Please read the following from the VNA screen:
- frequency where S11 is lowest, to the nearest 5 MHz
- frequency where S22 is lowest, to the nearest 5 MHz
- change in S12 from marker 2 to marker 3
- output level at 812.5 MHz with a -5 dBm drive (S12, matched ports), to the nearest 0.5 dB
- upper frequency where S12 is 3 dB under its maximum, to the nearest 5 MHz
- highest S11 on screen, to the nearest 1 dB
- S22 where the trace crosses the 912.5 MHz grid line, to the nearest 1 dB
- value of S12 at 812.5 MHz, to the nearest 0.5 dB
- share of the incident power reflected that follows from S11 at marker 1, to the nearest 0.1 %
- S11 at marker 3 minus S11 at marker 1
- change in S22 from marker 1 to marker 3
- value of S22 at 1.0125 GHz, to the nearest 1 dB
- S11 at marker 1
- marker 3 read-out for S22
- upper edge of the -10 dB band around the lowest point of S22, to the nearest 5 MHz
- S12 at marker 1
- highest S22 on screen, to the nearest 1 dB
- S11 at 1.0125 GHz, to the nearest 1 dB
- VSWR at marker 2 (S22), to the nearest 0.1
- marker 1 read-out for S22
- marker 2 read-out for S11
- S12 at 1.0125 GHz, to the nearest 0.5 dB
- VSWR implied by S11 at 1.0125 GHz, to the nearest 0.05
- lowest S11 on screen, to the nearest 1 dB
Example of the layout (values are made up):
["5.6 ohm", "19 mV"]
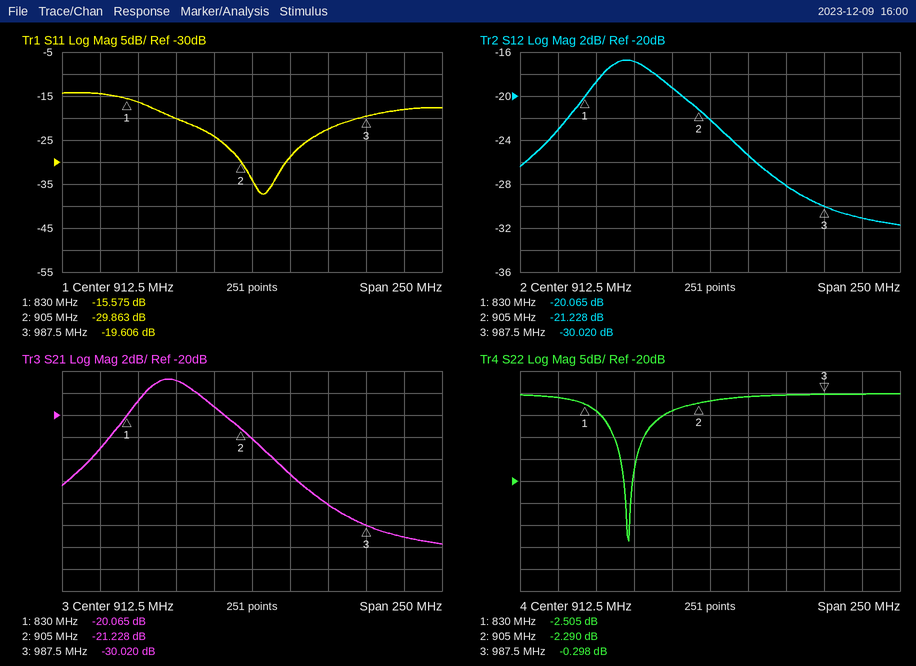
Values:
["920 MHz", "860 MHz", "-8.792 dB", "-28.0 dBm", "890 MHz", "-14 dB", "-2 dB", "-23.0 dB", "2.8 %", "-4.031 dB", "2.207 dB", "0 dB", "-15.575 dB", "-0.298 dB", "870 MHz", "-20.065 dB", "0 dB", "-18 dB", "7.6", "-2.505 dB", "-29.863 dB", "-31.0 dB", "1.30", "-37 dB"]
